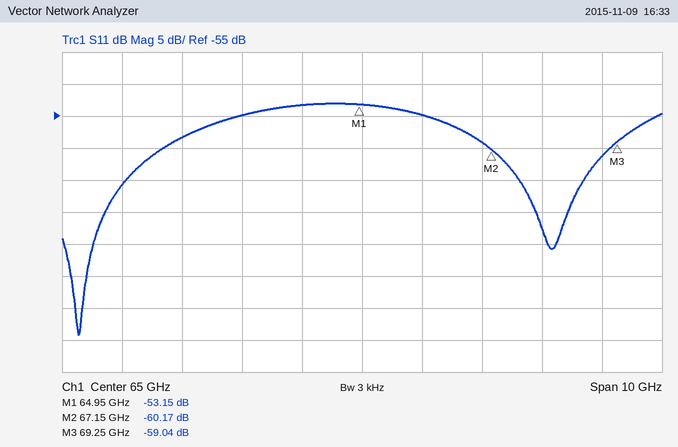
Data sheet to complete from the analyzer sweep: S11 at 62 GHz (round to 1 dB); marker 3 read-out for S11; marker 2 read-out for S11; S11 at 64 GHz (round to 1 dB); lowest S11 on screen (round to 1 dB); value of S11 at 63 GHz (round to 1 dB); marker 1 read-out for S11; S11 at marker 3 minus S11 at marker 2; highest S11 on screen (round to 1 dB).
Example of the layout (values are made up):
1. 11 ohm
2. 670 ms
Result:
1. -58 dB
2. -59.04 dB
3. -60.17 dB
4. -53 dB
5. -89 dB
6. -55 dB
7. -53.15 dB
8. 1.13 dB
9. -53 dB
